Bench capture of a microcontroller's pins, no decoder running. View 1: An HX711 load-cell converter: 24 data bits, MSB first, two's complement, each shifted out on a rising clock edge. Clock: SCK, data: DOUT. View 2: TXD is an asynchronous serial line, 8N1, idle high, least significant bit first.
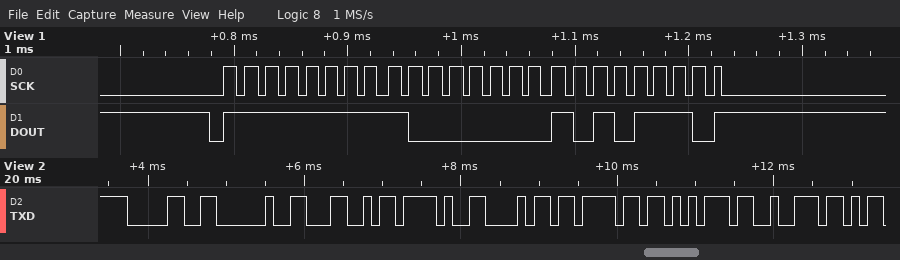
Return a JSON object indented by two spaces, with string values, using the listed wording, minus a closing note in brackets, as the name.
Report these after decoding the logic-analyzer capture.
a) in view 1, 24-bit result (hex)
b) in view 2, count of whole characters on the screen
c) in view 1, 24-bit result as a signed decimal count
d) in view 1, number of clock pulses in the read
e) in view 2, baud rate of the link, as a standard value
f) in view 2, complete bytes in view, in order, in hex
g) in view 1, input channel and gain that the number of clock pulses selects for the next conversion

{
  "in view 1, 24-bit result": "0xFF80AE",
  "in view 2, count of whole characters on the screen": "8",
  "in view 1, 24-bit result as a signed decimal count": "-32594",
  "in view 1, number of clock pulses in the read": "25",
  "in view 2, baud rate of the link, as a standard value": "9600 baud",
  "in view 2, complete bytes in view, in order, in hex": "30 20 4C 2F 68 6F 75 72",
  "in view 1, input channel and gain that the number of clock pulses selects for the next conversion": "channel A, gain 128"
}
